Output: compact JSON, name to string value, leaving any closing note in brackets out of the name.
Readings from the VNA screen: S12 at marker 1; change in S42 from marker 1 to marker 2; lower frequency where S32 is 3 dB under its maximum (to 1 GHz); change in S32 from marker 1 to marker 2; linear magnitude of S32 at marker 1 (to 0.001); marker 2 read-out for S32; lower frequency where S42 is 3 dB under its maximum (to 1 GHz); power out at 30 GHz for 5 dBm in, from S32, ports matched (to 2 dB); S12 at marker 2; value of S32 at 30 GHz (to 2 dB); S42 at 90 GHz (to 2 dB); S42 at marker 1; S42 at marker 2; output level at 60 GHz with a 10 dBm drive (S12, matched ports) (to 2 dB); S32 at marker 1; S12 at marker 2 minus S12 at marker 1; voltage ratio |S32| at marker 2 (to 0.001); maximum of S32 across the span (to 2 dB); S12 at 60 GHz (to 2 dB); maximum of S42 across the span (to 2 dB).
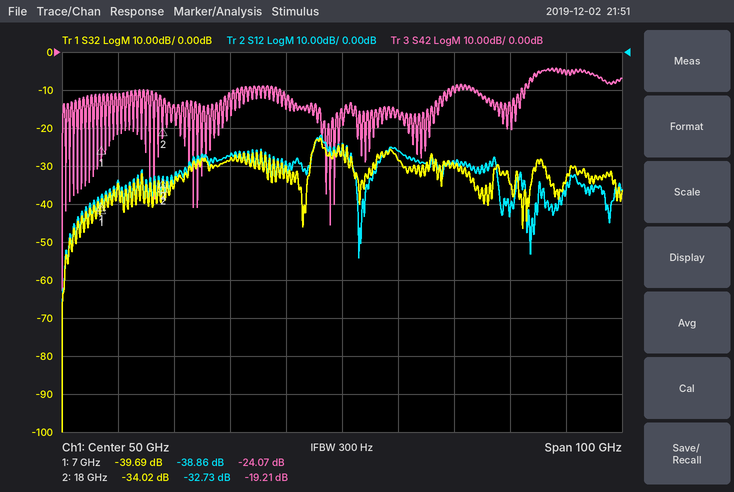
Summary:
{"S12 at marker 1": "-38.86 dB", "change in S42 from marker 1 to marker 2": "4.86 dB", "lower frequency where S32 is 3 dB under its maximum": "45 GHz", "change in S32 from marker 1 to marker 2": "5.67 dB", "linear magnitude of S32 at marker 1": "0.010", "marker 2 read-out for S32": "-34.02 dB", "lower frequency where S42 is 3 dB under its maximum": "84 GHz", "power out at 30 GHz for 5 dBm in, from S32, ports matched": "-24 dBm", "S12 at marker 2": "-32.73 dB", "value of S32 at 30 GHz": "-28 dB", "S42 at 90 GHz": "-6 dB", "S42 at marker 1": "-24.07 dB", "S42 at marker 2": "-19.21 dB", "output level at 60 GHz with a 10 dBm drive (S12, matched ports)": "-16 dBm", "S32 at marker 1": "-39.69 dB", "S12 at marker 2 minus S12 at marker 1": "6.13 dB", "voltage ratio |S32| at marker 2": "0.020", "maximum of S32 across the span": "-22 dB", "S12 at 60 GHz": "-26 dB", "maximum of S42 across the span": "-4 dB"}
